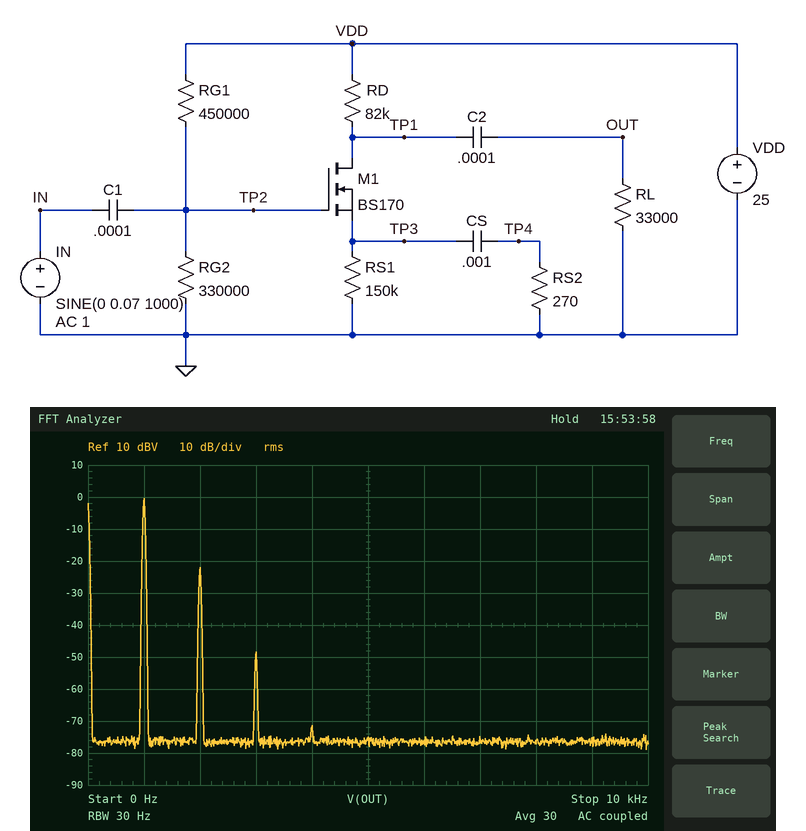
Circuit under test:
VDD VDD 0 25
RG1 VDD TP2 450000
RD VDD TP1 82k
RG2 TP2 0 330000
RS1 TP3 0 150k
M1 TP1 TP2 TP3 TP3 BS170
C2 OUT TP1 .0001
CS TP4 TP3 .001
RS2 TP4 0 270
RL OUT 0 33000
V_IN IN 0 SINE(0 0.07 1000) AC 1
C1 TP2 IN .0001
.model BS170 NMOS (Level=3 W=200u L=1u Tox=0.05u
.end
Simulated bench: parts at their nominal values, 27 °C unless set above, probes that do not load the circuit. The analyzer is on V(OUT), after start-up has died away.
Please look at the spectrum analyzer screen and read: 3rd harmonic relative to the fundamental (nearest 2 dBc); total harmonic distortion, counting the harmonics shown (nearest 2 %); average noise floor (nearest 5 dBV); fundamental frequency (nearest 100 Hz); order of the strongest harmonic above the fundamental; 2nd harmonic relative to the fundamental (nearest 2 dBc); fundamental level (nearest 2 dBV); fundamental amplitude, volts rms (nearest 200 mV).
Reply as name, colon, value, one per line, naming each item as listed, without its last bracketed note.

3rd harmonic relative to the fundamental: -48 dBc
total harmonic distortion, counting the harmonics shown: 8 %
average noise floor: -75 dBV
fundamental frequency: 1.0 kHz
order of the strongest harmonic above the fundamental: 2
2nd harmonic relative to the fundamental: -22 dBc
fundamental level: 0 dBV
fundamental amplitude, volts rms: 1.0 V
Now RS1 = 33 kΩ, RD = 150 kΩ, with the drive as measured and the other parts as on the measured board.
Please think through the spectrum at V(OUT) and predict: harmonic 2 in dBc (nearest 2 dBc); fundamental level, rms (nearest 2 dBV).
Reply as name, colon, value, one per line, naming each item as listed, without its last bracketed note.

harmonic 2 in dBc: -44 dBc
fundamental level, rms: -94 dBV
